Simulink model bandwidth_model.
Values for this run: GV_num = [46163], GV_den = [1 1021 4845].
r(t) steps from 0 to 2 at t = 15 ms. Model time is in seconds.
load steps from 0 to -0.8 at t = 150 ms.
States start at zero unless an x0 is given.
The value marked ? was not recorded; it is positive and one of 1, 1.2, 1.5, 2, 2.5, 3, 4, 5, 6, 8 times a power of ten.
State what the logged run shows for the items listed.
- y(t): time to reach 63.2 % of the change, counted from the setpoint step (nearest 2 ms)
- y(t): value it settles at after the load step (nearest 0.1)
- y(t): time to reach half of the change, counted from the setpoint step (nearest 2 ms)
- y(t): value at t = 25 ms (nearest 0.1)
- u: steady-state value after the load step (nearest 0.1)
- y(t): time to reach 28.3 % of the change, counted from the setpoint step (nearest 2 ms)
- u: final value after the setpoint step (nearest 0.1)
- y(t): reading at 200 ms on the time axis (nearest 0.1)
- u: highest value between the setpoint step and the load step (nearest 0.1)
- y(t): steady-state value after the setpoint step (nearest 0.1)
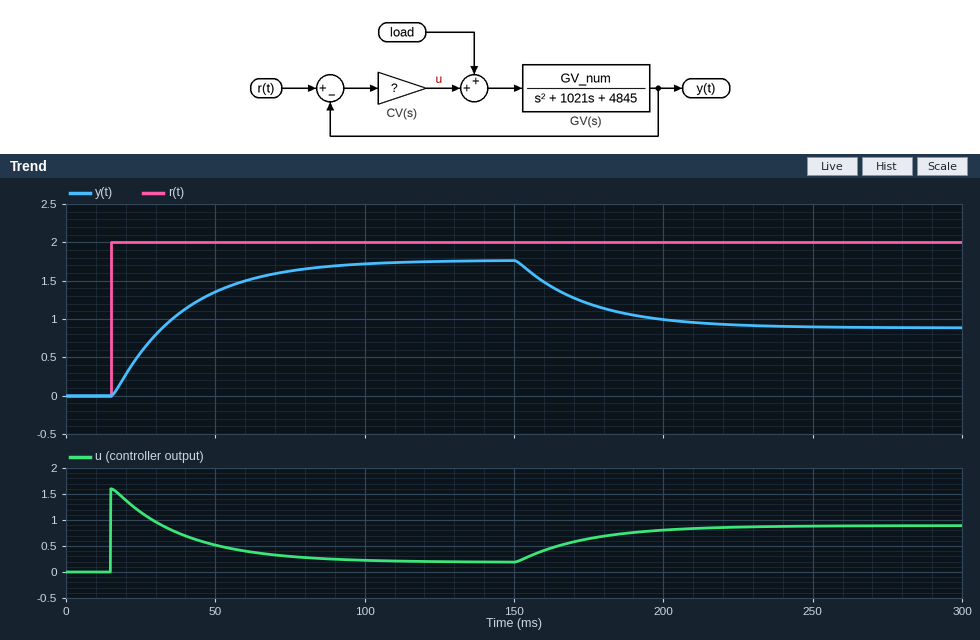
24 ms
0.9
18 ms
0.6
0.9
8 ms
0.2
1.0
1.6
1.8
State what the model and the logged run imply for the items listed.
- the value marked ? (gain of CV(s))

0.8
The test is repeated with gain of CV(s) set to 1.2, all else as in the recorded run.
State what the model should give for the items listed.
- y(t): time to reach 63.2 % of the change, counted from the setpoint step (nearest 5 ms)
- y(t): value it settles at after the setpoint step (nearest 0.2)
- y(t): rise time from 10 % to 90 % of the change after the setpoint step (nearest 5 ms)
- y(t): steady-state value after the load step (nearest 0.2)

15 ms
1.8
35 ms
1.2
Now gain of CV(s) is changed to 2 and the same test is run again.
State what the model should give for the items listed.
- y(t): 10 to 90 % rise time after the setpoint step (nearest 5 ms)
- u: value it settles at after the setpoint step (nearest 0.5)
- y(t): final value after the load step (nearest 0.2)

20 ms
0.0
1.6
